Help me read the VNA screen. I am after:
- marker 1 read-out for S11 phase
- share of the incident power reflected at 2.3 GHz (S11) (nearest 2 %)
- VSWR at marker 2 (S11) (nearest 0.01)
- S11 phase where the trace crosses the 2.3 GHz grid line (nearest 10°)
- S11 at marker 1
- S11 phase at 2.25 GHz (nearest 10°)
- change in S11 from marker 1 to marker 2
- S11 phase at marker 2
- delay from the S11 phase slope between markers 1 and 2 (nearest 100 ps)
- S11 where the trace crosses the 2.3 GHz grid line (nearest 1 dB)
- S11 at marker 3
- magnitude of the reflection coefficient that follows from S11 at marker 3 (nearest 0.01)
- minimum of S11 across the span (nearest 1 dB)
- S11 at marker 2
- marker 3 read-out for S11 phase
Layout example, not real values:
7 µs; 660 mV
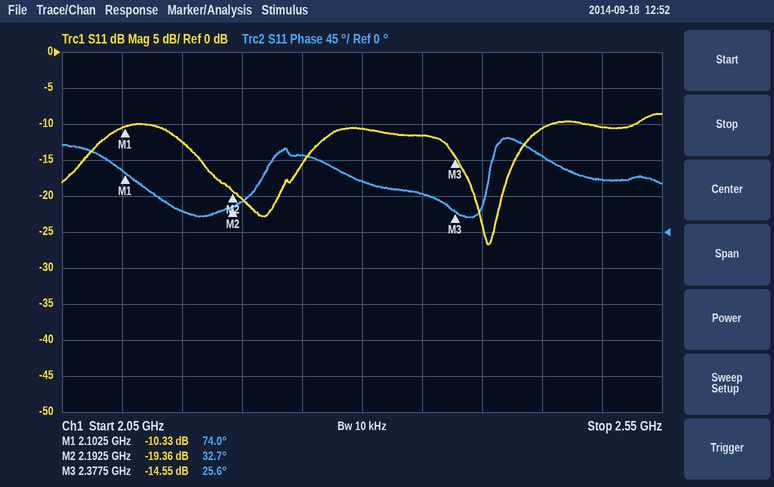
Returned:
74.0°; 8 %; 1.24; 60°; -10.33 dB; 100°; -9.03 dB; 32.7°; 1.3 ns; -11 dB; -14.55 dB; 0.19; -27 dB; -19.36 dB; 25.6°
